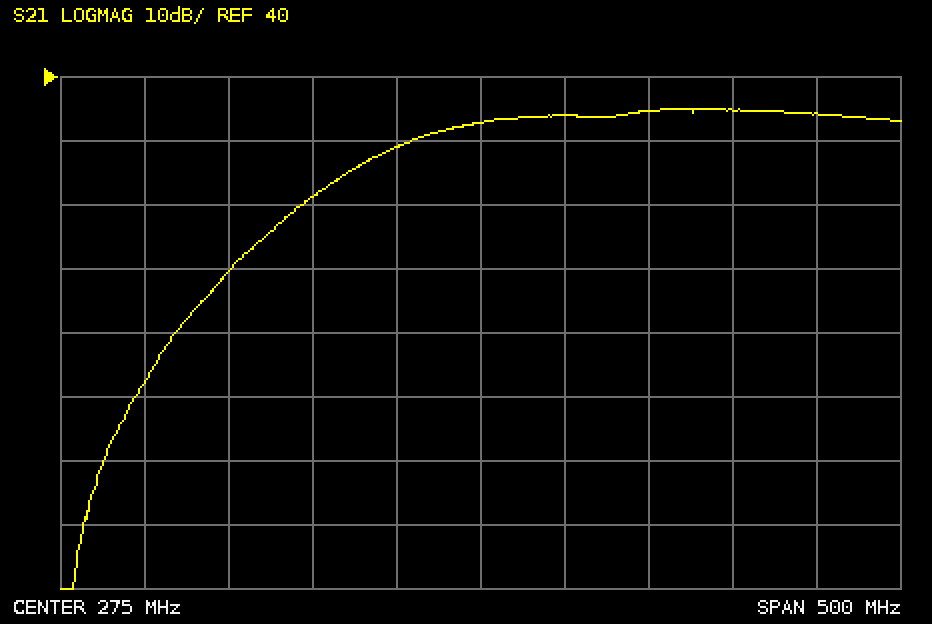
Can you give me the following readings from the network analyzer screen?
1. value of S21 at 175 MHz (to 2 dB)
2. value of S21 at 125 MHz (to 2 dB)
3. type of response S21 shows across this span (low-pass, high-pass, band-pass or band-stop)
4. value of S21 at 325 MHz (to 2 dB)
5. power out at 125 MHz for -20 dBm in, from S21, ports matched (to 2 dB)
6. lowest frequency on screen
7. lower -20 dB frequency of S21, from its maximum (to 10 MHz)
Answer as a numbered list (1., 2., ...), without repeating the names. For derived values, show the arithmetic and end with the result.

1. 22 dB
2. 10 dB
3. high-pass
4. 34 dB
5. -20 dBm + (10 dB) = -10 dBm
6. 25 MHz
7. 150 MHz
